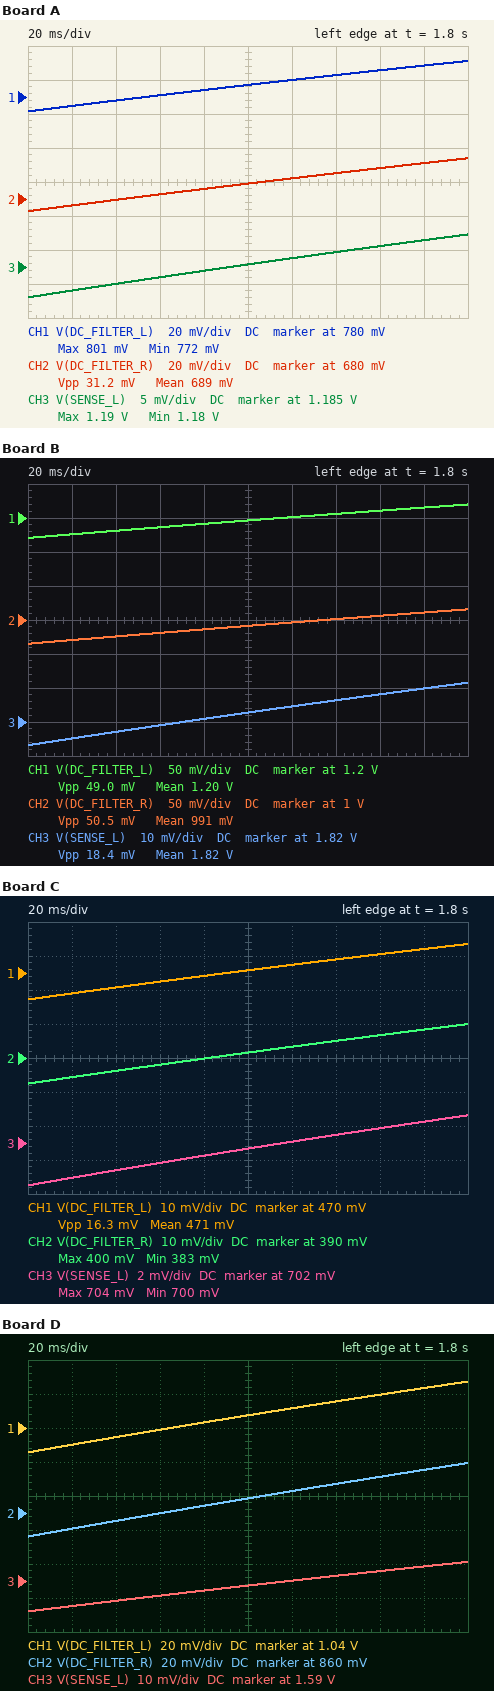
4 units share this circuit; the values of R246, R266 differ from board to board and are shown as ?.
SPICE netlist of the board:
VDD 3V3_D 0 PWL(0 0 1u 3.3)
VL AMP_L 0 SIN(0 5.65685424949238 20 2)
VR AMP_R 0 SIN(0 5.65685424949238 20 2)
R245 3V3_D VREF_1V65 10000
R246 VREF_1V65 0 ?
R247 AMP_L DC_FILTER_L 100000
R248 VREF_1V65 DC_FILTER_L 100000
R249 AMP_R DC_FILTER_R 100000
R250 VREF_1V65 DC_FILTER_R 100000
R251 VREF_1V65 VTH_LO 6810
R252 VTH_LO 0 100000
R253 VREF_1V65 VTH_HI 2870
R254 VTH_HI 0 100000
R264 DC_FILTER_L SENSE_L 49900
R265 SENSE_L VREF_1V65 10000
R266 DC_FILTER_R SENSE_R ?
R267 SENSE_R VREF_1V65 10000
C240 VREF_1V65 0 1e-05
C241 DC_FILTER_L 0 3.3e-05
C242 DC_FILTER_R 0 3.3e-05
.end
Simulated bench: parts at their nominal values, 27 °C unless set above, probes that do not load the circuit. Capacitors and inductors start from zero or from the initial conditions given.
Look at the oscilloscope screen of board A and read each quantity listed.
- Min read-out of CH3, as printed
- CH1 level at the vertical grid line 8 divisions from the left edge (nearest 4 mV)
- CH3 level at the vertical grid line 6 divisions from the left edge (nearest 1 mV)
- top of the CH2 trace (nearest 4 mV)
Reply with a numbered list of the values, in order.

1. 1.18 V
2. 796 mV
3. 1.186 V
4. 704 mV
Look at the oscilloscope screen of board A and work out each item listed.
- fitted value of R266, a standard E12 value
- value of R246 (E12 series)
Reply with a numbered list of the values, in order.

1. 82 kΩ
2. 8.2 kΩ
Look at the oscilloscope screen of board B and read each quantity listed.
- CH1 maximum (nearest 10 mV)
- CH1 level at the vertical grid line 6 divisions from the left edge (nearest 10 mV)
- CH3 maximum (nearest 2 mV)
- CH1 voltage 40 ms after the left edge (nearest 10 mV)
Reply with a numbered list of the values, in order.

1. 1.22 V
2. 1.20 V
3. 1.832 V
4. 1.18 V
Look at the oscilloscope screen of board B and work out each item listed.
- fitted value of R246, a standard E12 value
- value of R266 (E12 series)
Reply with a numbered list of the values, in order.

1. 33 kΩ
2. 100 kΩ
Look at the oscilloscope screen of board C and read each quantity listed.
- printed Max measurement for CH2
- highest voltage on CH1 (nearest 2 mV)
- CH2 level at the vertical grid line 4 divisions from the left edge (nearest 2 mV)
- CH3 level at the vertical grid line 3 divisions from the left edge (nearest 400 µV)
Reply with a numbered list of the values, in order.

1. 400 mV
2. 478 mV
3. 390 mV
4. 700.8 mV
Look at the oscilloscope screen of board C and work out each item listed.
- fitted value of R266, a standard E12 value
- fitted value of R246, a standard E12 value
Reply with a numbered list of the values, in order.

1. 100 kΩ
2. 3.3 kΩ
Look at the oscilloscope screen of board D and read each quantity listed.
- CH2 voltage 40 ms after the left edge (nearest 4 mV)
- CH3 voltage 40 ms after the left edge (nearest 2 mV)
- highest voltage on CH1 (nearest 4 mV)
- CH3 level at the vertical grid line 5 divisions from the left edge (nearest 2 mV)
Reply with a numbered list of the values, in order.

1. 856 mV
2. 1.584 V
3. 1.068 V
4. 1.588 V
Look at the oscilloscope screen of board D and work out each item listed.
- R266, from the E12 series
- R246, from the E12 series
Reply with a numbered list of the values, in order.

1. 100 kΩ
2. 18 kΩ
